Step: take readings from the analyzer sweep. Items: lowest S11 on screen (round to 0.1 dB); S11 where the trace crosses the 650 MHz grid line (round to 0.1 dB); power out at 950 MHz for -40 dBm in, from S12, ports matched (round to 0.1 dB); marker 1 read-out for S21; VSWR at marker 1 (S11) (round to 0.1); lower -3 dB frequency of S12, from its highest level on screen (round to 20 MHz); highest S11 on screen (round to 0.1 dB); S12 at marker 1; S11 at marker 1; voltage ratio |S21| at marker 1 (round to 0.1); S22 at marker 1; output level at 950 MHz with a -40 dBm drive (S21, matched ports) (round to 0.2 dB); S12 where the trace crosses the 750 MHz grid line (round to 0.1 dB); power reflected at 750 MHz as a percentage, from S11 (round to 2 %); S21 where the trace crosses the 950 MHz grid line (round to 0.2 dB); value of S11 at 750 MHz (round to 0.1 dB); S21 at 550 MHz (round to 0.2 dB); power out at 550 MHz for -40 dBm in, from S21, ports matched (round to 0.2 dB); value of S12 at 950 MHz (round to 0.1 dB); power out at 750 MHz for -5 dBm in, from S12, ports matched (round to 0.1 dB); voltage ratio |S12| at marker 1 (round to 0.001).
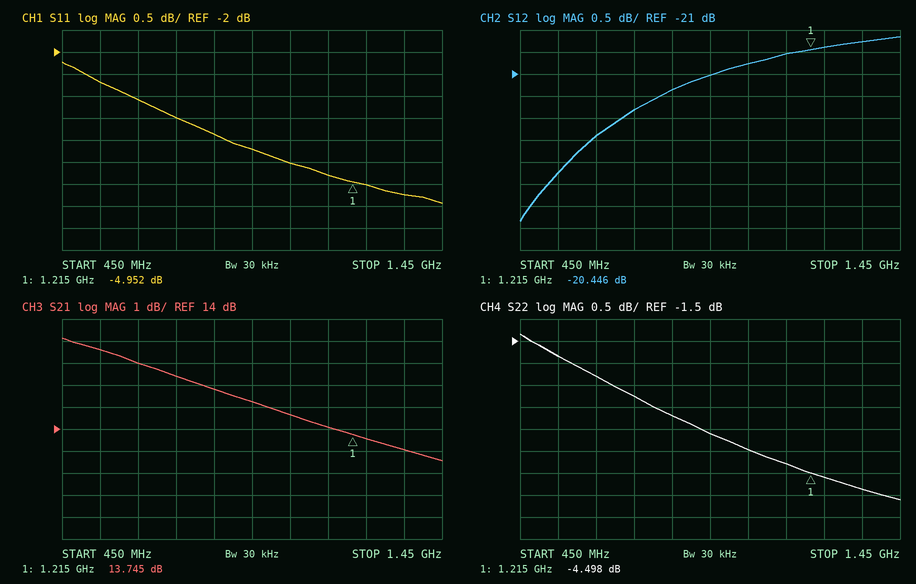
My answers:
-5.4 dB
-3.1 dB
-61.0 dBm
13.745 dB
3.6
560 MHz
-2.2 dB
-20.446 dB
-4.952 dB
4.9
-4.498 dB
-24.8 dBm
-21.8 dB
44 %
15.2 dB
-3.5 dB
17.6 dB
-22.4 dBm
-21.0 dB
-26.8 dBm
0.095
